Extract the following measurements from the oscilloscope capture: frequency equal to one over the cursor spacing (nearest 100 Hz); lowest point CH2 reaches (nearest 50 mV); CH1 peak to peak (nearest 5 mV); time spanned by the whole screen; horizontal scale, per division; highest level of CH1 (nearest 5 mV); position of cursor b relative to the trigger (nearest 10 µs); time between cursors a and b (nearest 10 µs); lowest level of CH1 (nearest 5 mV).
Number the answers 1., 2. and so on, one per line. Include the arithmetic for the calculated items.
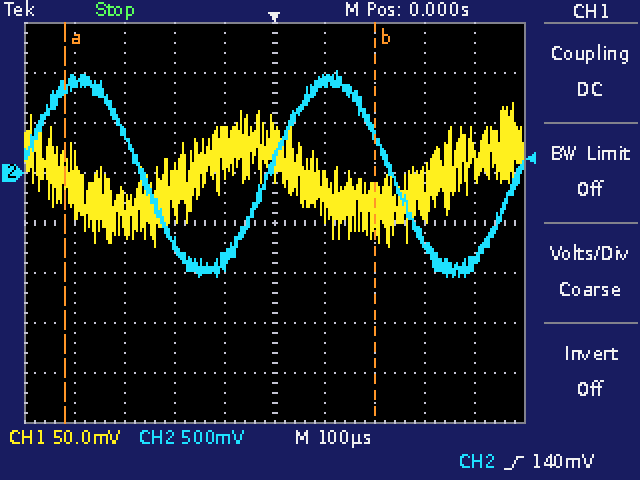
1. 1 / 620 µs ≈ 1.6 kHz
2. -1.05 V
3. 70 mV − (-75 mV) = 145 mV
4. 1 ms
5. 100 µs
6. 70 mV
7. +200 µs
8. 620 µs
9. -75 mV
